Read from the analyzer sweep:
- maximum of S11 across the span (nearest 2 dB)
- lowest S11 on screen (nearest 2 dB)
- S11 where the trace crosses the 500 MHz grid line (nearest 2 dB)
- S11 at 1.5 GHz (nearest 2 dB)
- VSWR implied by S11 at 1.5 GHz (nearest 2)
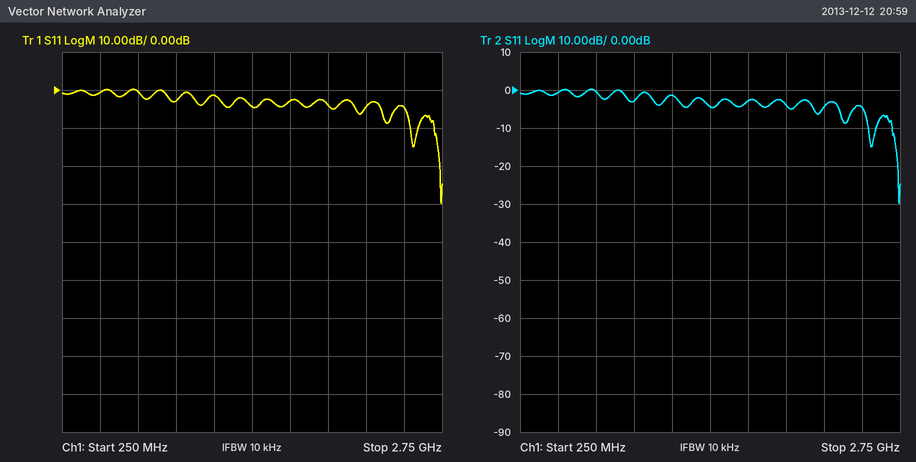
0 dB
-30 dB
0 dB
-4 dB
4
